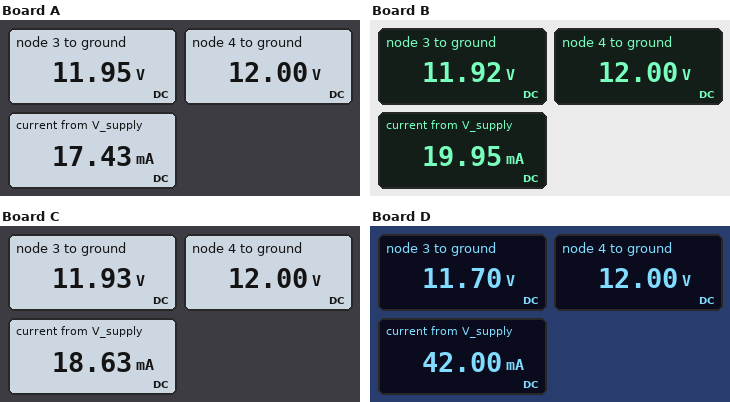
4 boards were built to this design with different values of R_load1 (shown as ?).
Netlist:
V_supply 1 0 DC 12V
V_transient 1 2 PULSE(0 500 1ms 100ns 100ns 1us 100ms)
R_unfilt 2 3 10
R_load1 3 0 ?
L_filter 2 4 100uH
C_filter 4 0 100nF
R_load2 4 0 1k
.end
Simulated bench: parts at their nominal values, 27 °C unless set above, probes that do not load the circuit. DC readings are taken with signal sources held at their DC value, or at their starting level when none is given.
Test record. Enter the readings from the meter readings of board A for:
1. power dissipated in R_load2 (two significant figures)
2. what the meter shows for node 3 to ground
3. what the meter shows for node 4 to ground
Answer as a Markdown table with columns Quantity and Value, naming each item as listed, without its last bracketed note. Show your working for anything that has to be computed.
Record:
| Quantity | Value |
|---|---|
| power dissipated in R_load2 | (12 V)^2 / 1 kΩ = 140 mW |
| what the meter shows for node 3 to ground | 11.95 V |
| what the meter shows for node 4 to ground | 12.00 V |
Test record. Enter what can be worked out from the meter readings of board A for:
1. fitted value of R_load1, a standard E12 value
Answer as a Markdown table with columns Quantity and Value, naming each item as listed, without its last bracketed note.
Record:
| Quantity | Value |
|---|---|
| fitted value of R_load1, a standard E12 value | 2.2 kΩ |
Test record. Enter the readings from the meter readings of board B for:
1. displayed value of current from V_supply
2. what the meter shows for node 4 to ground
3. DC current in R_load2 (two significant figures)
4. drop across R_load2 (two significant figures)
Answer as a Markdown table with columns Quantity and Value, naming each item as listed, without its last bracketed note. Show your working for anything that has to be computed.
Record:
| Quantity | Value |
|---|---|
| displayed value of current from V_supply | 19.95 mA |
| what the meter shows for node 4 to ground | 12.00 V |
| DC current in R_load2 | (12 V) / 1 kΩ = 12 mA |
| drop across R_load2 | 12 V = 12 V |
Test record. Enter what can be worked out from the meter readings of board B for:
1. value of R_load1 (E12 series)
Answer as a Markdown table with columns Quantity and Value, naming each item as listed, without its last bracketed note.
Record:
| Quantity | Value |
|---|---|
| value of R_load1 | 1.5 kΩ |
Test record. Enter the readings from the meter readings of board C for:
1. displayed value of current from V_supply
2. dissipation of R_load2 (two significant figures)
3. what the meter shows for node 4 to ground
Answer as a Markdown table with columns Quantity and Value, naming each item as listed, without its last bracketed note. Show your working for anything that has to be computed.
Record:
| Quantity | Value |
|---|---|
| displayed value of current from V_supply | 18.63 mA |
| dissipation of R_load2 | (12 V)^2 / 1 kΩ = 140 mW |
| what the meter shows for node 4 to ground | 12.00 V |
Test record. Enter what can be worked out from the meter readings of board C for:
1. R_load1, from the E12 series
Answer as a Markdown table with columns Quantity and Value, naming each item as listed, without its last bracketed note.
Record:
| Quantity | Value |
|---|---|
| R_load1, from the E12 series | 1.8 kΩ |
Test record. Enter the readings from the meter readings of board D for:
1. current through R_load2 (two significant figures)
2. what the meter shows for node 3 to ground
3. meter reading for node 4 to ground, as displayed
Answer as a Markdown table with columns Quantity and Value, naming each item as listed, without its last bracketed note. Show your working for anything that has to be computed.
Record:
| Quantity | Value |
|---|---|
| current through R_load2 | (12 V) / 1 kΩ = 12 mA |
| what the meter shows for node 3 to ground | 11.70 V |
| meter reading for node 4 to ground, as displayed | 12.00 V |
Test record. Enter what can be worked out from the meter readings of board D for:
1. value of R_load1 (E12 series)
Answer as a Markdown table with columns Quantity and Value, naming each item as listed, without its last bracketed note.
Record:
| Quantity | Value |
|---|---|
| value of R_load1 | 390 Ω |
